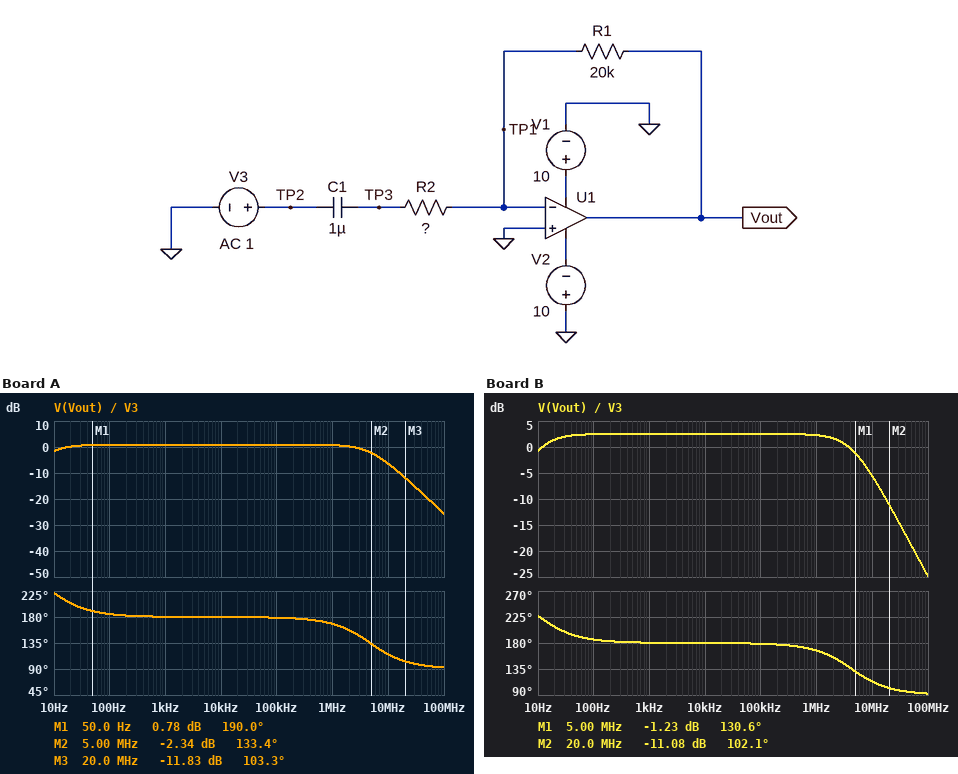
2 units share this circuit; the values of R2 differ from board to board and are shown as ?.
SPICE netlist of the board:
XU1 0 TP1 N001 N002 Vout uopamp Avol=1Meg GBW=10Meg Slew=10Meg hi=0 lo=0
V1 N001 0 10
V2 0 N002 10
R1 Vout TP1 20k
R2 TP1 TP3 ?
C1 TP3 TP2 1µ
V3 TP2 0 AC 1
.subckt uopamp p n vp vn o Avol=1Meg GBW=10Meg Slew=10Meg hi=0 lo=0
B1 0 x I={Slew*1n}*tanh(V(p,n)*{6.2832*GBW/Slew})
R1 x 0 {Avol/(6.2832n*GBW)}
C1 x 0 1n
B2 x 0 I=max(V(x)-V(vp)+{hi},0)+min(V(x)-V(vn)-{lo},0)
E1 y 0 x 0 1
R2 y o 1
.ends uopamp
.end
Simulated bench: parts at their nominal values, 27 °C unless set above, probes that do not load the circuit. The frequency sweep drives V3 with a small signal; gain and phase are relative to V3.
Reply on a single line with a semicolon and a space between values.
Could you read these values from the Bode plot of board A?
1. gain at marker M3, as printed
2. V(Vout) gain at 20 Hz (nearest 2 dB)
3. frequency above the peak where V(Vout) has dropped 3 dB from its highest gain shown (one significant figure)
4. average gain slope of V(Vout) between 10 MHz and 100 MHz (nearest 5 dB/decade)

-11.83 dB; 0 dB; 5 MHz; -20 dB/decade
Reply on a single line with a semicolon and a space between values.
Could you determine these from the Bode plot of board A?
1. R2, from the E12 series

18 kΩ
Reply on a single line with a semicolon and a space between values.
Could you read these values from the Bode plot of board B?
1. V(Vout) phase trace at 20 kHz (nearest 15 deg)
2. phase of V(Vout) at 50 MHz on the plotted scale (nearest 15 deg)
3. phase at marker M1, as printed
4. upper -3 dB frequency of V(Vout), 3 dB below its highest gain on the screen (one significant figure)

180 deg; 90 deg; 130.6 deg; 4 MHz
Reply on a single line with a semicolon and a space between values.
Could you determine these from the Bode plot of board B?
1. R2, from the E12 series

15 kΩ
